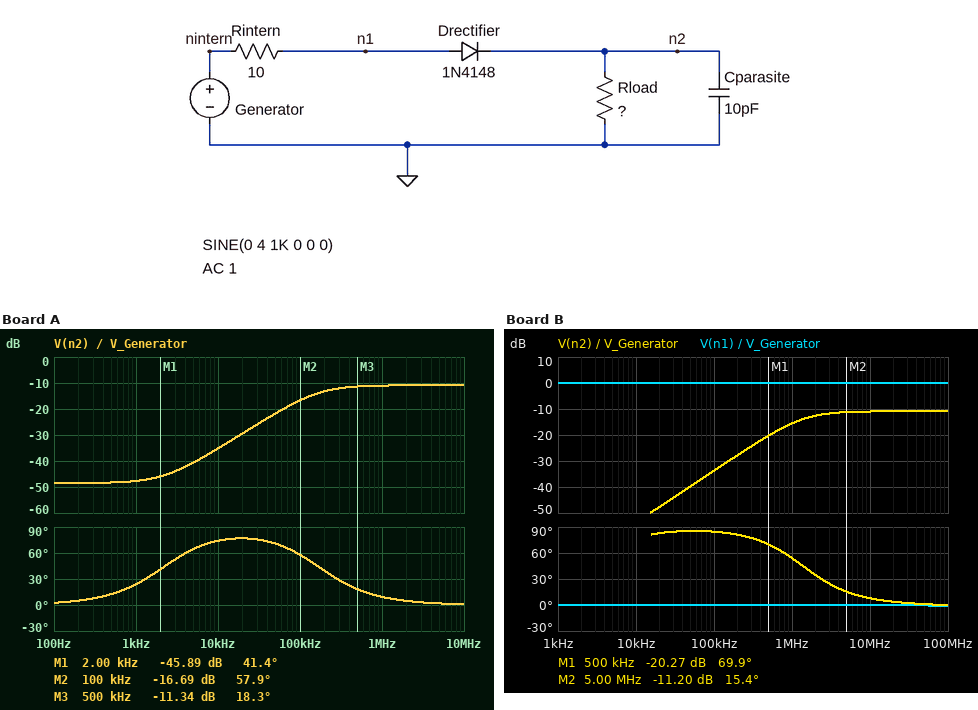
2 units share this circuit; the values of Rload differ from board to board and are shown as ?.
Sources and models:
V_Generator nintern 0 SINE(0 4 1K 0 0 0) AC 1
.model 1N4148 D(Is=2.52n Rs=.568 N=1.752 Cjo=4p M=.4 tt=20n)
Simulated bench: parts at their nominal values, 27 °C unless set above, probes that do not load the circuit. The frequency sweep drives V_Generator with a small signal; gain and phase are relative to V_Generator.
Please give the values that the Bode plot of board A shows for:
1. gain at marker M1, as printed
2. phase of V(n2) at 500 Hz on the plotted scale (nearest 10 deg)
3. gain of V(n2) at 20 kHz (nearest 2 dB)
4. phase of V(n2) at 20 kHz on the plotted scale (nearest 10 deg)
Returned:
-45.89 dB
10 deg
-30 dB
80 deg
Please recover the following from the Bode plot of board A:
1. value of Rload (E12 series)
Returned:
68 kΩ
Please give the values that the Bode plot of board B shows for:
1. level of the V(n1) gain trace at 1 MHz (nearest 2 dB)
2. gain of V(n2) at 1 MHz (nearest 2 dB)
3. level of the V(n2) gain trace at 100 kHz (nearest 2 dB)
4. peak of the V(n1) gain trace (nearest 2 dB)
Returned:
0 dB
-16 dB
-34 dB
0 dB
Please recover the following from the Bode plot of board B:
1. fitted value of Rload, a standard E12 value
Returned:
8.2 kΩ
